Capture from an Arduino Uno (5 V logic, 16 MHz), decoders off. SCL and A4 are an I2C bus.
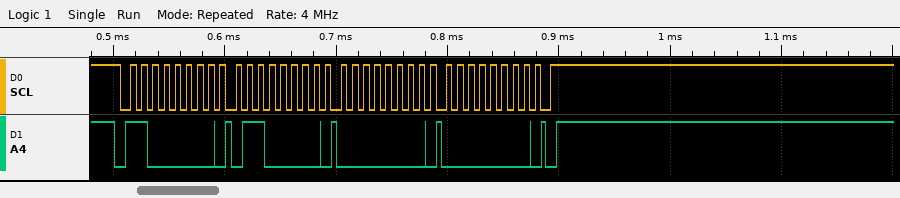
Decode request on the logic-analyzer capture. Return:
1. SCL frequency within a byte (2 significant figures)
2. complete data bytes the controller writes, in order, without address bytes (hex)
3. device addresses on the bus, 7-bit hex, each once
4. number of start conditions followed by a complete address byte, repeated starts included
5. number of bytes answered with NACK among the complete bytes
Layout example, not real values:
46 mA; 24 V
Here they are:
100 kHz; 60 00 00; 0x60; 1; 0
